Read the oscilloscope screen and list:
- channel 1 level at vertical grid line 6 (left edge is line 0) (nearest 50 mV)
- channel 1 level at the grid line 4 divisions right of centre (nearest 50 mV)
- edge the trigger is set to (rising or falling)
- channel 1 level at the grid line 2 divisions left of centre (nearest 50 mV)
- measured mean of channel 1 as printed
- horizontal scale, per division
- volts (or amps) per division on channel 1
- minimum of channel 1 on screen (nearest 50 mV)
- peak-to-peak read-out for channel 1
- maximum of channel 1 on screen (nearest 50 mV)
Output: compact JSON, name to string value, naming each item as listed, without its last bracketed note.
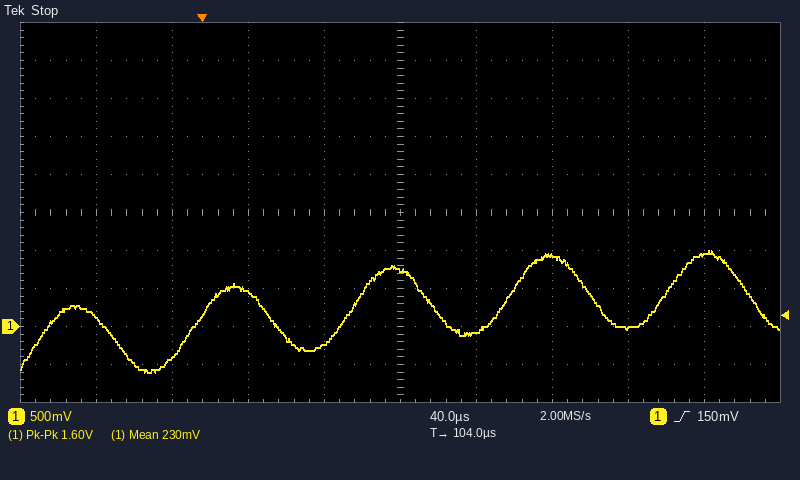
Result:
{"channel 1 level at vertical grid line 6 (left edge is line 0)": "-50 mV", "channel 1 level at the grid line 4 divisions right of centre": "950 mV", "edge the trigger is set to": "rising", "channel 1 level at the grid line 2 divisions left of centre": "450 mV", "measured mean of channel 1 as printed": "230 mV", "horizontal scale, per division": "40 µs", "volts (or amps) per division on channel 1": "500 mV", "minimum of channel 1 on screen": "-600 mV", "peak-to-peak read-out for channel 1": "1.60 V", "maximum of channel 1 on screen": "1.00 V"}
